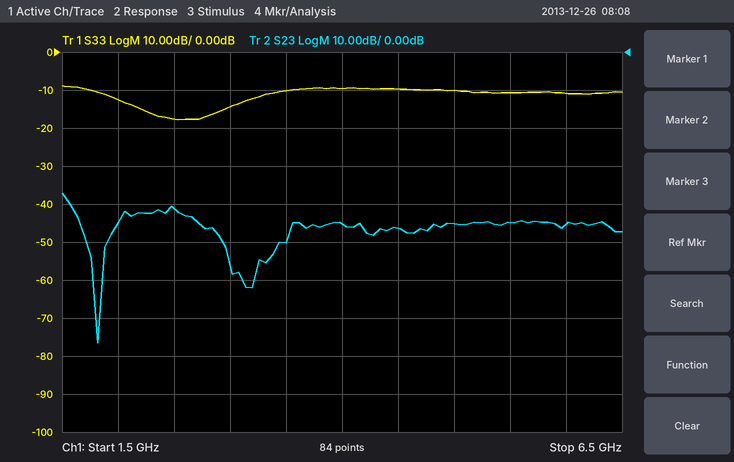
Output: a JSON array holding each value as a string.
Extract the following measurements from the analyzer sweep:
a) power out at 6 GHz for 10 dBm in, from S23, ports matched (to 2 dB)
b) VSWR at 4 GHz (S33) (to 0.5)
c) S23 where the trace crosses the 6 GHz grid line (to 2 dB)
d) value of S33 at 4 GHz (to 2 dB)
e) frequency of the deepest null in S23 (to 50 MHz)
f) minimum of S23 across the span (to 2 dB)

["-36 dBm", "2.0", "-46 dB", "-10 dB", "1.80 GHz", "-76 dB"]
